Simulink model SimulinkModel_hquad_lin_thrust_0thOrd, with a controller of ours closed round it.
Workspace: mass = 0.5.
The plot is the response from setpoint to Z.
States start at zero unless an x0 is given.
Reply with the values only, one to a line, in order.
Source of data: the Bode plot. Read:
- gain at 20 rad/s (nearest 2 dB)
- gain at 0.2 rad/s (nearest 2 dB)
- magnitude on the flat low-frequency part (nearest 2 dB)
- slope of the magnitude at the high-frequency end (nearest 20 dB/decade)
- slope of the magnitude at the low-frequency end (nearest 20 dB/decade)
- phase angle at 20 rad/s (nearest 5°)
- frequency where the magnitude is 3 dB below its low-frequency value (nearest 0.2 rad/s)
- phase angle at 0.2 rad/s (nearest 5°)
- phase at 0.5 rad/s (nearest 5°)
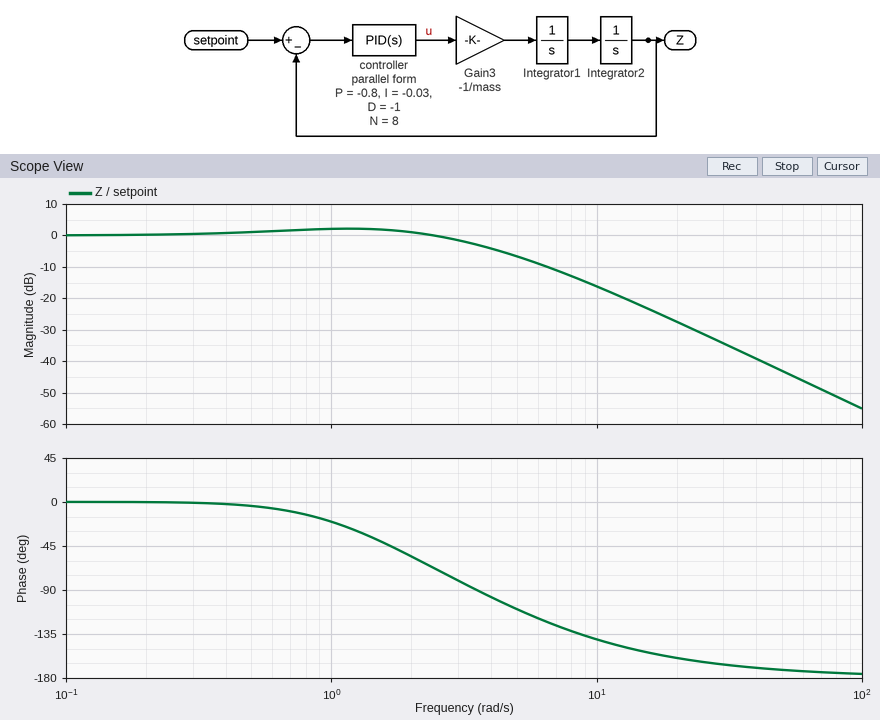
-28 dB
0 dB
0 dB
-40 dB/decade
0 dB/decade
-160°
3.6 rad/s
0°
-5°
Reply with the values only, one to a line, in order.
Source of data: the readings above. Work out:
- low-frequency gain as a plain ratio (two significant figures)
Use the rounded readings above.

1.0
